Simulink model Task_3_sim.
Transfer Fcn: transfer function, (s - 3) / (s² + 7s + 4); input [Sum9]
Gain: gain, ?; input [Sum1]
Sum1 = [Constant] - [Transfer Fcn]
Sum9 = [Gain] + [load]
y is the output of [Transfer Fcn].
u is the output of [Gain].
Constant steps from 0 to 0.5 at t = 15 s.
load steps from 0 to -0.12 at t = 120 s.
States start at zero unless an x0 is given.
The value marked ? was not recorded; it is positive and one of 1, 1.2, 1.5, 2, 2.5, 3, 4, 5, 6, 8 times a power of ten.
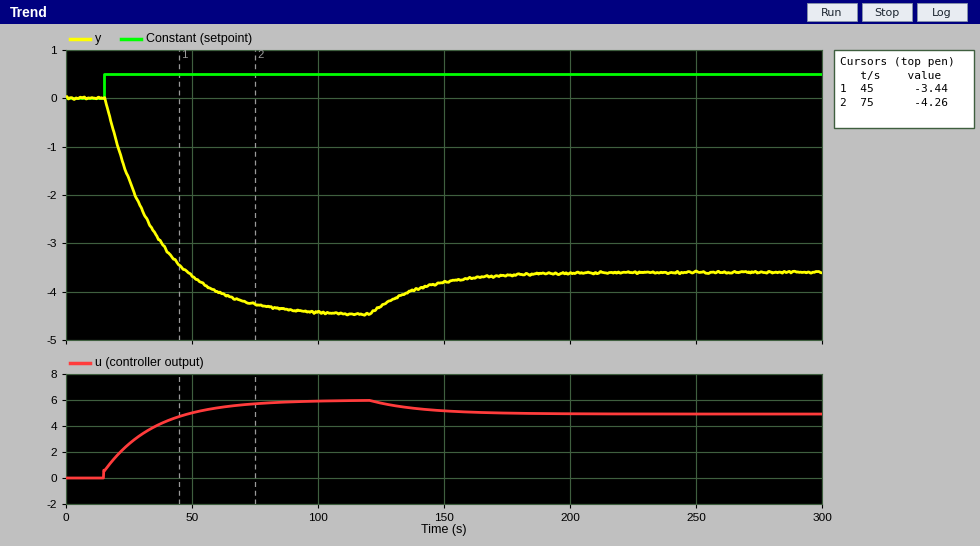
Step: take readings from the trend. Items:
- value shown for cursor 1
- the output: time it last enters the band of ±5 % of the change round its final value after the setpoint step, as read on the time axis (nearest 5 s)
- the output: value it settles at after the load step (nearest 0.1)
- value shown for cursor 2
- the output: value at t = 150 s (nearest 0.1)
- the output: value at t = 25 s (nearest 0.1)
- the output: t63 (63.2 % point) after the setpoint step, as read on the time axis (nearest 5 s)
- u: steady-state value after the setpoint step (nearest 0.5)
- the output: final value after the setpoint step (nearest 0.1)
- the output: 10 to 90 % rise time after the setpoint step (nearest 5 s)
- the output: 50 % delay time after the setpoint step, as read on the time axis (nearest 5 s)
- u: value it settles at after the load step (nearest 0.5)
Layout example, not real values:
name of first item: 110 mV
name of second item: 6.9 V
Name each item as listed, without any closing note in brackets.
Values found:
value shown for cursor 1: -3.44
the output: time it last enters the band of ±5 % of the change round its final value after the setpoint step, as read on the time axis: 75 s
the output: value it settles at after the load step: -3.6
value shown for cursor 2: -4.26
the output: value at t = 150 s: -3.8
the output: value at t = 25 s: -1.7
the output: t63 (63.2 % point) after the setpoint step, as read on the time axis: 35 s
u: steady-state value after the setpoint step: 6.0
the output: final value after the setpoint step: -4.5
the output: 10 to 90 % rise time after the setpoint step: 45 s
the output: 50 % delay time after the setpoint step, as read on the time axis: 30 s
u: value it settles at after the load step: 5.0
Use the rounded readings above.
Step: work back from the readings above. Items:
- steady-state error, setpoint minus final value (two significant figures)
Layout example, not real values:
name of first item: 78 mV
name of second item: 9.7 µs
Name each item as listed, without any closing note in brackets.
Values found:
steady-state error, setpoint minus final value: 5.0
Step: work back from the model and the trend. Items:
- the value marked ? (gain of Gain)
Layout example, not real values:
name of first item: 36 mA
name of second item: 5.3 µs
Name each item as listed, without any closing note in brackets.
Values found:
the value marked ?: 1.2
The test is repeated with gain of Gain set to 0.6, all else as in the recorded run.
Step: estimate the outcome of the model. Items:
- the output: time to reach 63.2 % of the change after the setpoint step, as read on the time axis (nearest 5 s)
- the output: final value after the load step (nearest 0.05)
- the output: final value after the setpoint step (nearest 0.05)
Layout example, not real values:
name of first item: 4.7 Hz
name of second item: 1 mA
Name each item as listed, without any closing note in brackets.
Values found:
the output: time to reach 63.2 % of the change after the setpoint step, as read on the time axis: 20 s
the output: final value after the load step: -0.25
the output: final value after the setpoint step: -0.40
